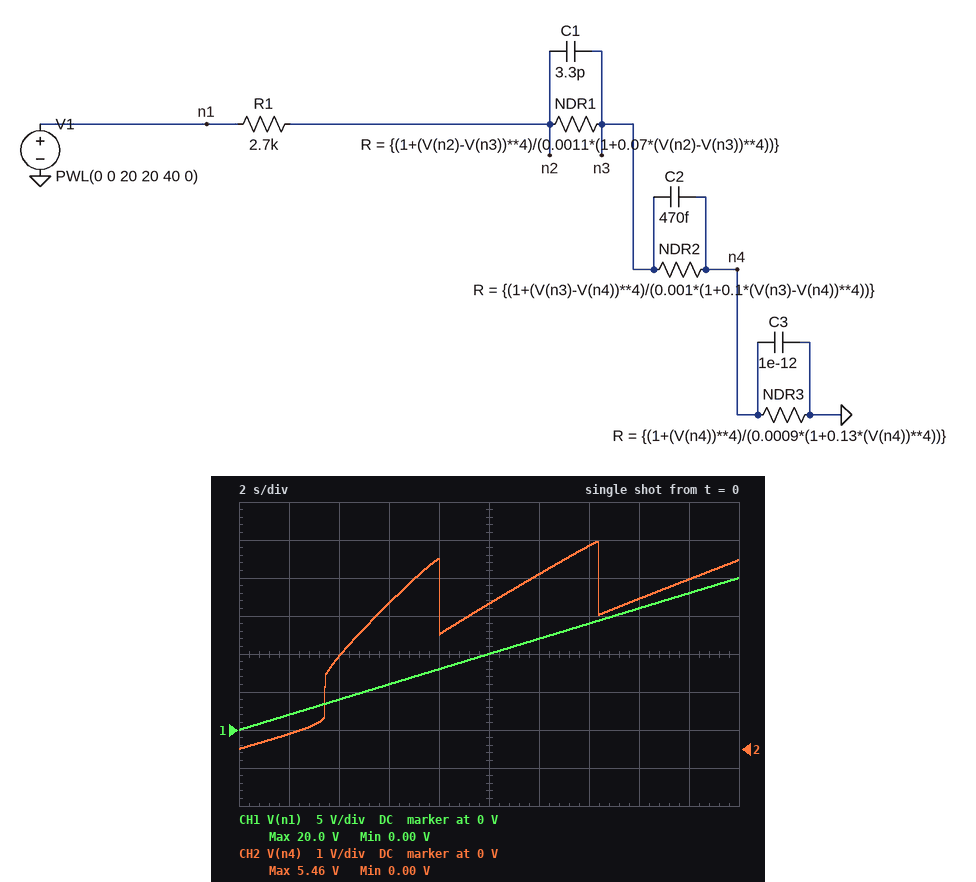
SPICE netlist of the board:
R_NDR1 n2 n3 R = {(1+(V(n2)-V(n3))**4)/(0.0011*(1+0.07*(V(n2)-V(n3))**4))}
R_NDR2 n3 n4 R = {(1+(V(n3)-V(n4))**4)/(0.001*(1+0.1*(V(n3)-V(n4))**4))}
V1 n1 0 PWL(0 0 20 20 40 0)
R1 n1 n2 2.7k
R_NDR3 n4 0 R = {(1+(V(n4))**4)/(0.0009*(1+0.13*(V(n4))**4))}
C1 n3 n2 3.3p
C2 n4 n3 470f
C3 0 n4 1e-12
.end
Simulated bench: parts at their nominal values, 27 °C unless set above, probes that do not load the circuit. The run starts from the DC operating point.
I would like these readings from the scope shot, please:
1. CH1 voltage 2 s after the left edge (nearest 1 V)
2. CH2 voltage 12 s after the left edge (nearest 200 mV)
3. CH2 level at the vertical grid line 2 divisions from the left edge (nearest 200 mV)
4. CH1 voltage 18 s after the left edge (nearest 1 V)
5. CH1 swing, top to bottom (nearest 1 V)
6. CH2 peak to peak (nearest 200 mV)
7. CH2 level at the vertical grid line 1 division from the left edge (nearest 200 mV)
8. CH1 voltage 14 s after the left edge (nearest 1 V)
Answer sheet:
2 V
4.6 V
2.4 V
18 V
20 V
5.4 V
400 mV
14 V
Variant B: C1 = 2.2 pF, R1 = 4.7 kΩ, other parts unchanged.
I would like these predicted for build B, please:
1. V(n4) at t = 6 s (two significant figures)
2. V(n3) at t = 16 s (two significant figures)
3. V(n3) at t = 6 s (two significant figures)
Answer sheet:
3.3 V
8.1 V
3.7 V
